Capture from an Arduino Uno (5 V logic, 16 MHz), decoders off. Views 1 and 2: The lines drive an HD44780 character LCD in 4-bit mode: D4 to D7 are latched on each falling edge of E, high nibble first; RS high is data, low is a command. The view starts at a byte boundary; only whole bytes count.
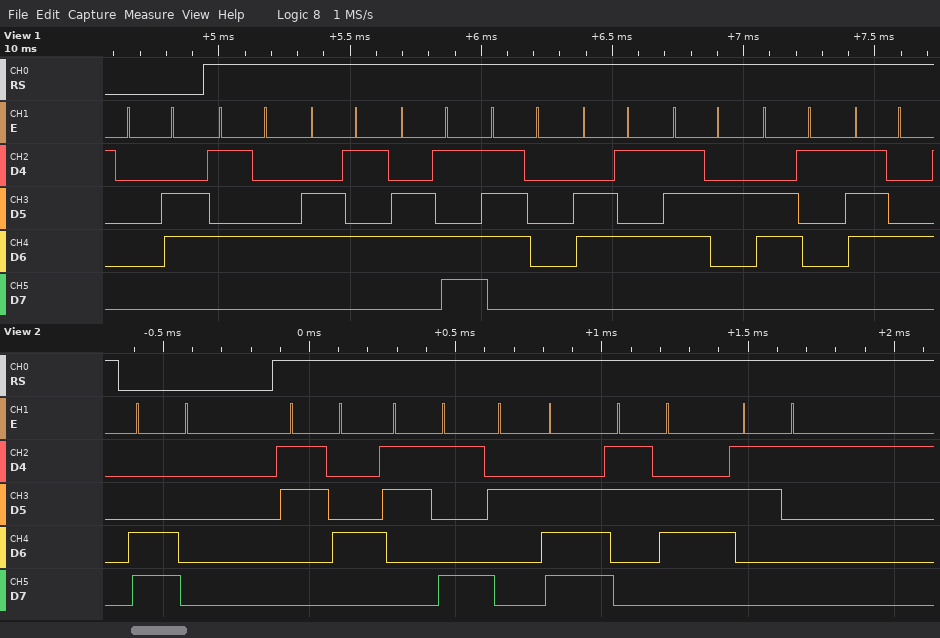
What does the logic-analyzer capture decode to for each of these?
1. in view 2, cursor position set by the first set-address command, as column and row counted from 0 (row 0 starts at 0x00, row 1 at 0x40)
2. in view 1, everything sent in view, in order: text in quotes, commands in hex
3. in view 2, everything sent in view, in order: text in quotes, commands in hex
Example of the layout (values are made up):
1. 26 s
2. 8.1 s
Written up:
1. column 0, row 1
2. 0x06 "Temperat"
3. 0xC0 "49.61"
